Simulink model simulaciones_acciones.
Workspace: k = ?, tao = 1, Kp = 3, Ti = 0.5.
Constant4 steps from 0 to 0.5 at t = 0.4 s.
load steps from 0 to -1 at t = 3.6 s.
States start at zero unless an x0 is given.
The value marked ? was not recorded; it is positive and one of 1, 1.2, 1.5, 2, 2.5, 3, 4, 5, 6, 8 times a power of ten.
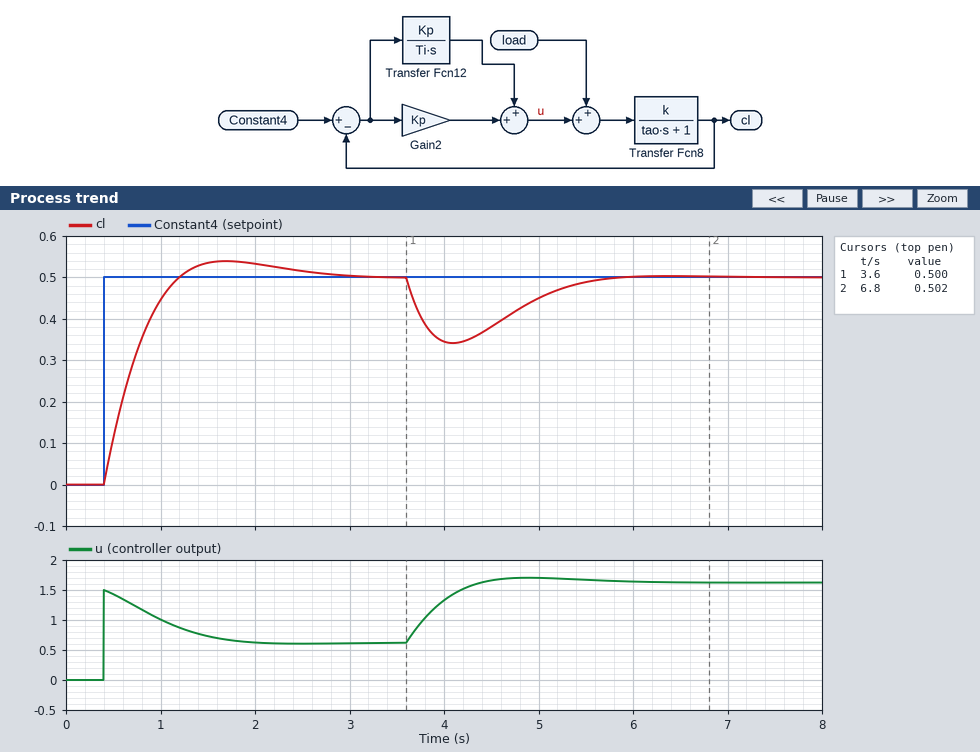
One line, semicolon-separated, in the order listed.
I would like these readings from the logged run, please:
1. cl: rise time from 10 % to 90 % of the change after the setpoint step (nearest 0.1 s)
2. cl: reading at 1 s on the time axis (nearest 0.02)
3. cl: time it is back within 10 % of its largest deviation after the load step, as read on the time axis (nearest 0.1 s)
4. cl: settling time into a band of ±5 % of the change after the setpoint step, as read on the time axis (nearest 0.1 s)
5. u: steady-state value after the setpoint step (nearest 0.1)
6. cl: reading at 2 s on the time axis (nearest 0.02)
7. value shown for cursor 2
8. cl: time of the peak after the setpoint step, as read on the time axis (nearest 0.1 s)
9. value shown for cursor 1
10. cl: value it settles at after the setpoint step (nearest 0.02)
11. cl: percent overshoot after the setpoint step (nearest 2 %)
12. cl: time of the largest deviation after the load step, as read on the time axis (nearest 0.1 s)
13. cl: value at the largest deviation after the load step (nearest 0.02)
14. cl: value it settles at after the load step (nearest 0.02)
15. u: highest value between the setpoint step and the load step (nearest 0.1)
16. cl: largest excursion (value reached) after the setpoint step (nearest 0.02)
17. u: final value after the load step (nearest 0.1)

0.6 s; 0.44; 5.4 s; 2.2 s; 0.6; 0.54; 0.502; 1.7 s; 0.500; 0.50; 8 %; 4.1 s; 0.34; 0.50; 1.5; 0.54; 1.6
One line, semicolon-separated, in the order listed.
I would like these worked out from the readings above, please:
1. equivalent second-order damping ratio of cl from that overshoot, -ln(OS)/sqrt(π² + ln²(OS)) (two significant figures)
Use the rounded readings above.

0.63
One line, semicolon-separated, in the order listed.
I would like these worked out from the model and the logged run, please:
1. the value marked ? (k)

0.8
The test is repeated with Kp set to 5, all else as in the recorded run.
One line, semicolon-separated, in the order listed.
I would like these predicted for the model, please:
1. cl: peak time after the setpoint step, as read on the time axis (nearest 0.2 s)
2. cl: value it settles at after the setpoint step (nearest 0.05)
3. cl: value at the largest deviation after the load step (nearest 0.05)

1.4 s; 0.50; 0.40
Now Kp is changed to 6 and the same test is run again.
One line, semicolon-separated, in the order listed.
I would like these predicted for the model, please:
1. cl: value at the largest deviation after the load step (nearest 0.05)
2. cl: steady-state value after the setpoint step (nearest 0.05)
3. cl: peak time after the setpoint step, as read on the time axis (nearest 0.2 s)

0.40; 0.50; 1.2 s
